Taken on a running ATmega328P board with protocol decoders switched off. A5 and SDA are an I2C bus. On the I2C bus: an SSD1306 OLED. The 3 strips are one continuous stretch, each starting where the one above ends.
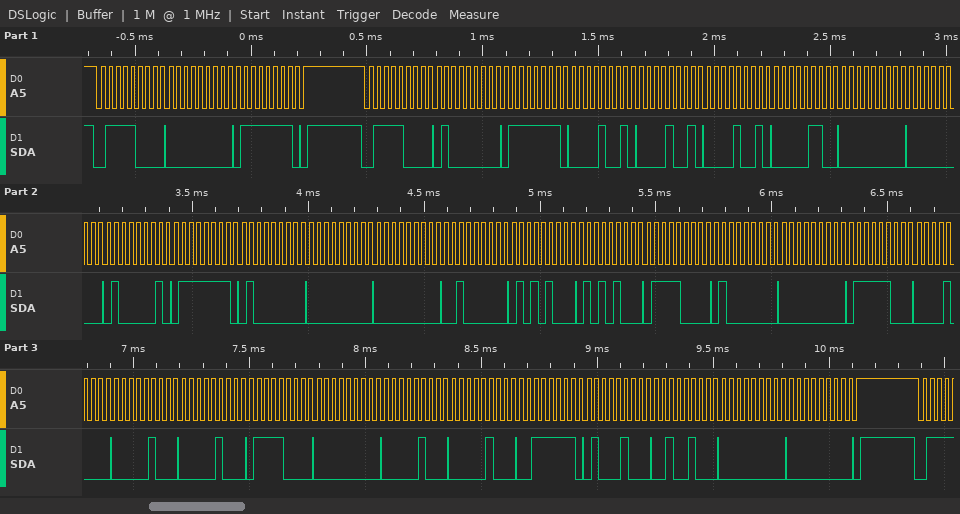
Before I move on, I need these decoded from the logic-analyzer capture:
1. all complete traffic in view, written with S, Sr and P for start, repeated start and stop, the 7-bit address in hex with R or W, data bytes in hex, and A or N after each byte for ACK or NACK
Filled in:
S 3CW A 00 A 7F A P S 3CW A 40 A 7F A 09 A 09 A 09 A 06 A 00 A 00 A 41 A 7F A 40 A 00 A 00 A 20 A 54 A 54 A 78 A 40 A 00 A 7C A 08 A 04 A 04 A 78 A 00 A 04 A 04 A 3F A 44 A 24 A 00 A 00 A P
